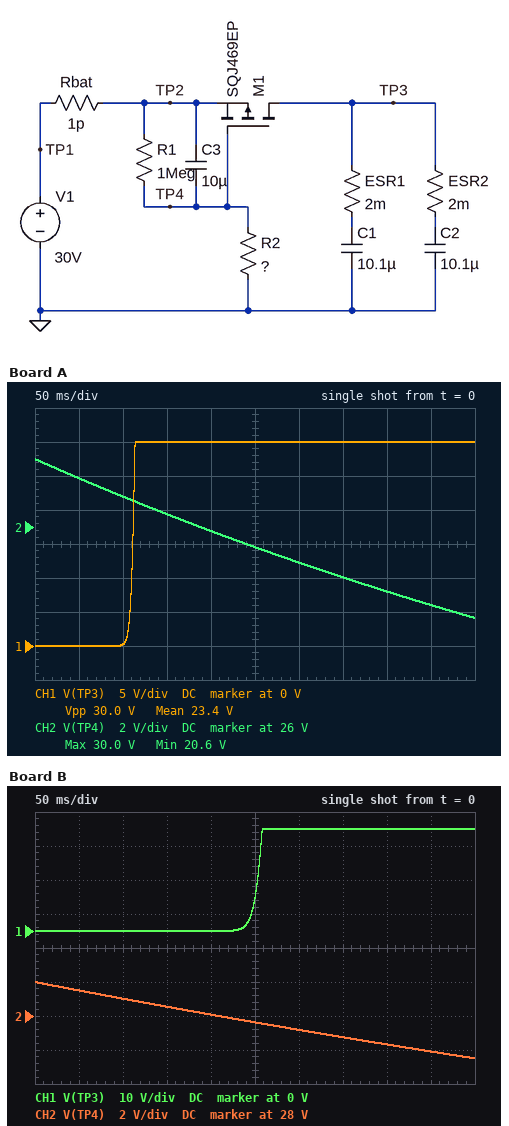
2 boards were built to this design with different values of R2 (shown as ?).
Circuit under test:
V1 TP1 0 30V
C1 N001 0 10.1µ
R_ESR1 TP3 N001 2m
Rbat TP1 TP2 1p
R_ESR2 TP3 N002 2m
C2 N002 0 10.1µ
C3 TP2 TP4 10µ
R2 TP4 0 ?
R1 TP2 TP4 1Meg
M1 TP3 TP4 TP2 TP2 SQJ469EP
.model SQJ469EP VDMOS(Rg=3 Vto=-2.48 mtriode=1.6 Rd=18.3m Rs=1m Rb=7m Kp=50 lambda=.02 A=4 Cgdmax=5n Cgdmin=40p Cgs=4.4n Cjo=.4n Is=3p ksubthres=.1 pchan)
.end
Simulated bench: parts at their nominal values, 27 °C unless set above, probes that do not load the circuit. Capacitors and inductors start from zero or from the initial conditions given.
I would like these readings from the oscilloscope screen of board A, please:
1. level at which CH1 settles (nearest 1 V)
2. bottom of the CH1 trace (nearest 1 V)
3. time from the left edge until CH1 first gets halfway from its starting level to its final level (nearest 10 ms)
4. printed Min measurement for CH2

30 V
0 V
110 ms
20.6 V
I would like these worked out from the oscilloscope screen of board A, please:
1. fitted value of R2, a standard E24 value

130 kΩ
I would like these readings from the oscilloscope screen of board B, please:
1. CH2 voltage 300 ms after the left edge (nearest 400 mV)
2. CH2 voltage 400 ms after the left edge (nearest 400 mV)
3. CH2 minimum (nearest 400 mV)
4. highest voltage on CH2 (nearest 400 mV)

27.2 V
26.4 V
25.6 V
30.0 V
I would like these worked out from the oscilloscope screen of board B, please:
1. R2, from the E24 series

300 kΩ
